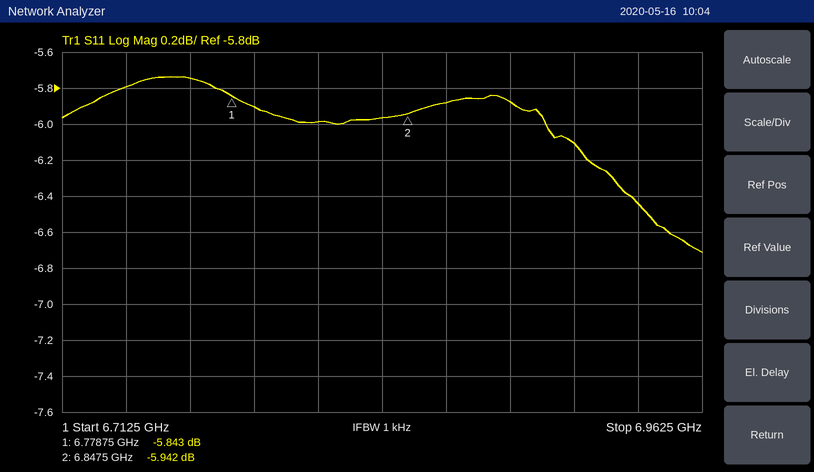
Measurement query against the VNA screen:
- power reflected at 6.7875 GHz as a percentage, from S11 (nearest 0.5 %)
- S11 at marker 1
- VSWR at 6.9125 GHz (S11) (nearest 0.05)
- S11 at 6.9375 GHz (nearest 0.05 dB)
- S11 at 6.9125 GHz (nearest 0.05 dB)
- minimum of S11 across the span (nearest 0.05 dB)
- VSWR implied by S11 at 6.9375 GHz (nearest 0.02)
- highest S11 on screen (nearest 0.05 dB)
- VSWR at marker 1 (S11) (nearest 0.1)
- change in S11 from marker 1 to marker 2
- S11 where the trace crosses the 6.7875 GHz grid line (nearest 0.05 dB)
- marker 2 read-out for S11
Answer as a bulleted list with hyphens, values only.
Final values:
- 25.5 %
- -5.843 dB
- 2.95
- -6.45 dB
- -6.10 dB
- -6.70 dB
- 2.82
- -5.75 dB
- 3.1
- -0.099 dB
- -5.90 dB
- -5.942 dB
